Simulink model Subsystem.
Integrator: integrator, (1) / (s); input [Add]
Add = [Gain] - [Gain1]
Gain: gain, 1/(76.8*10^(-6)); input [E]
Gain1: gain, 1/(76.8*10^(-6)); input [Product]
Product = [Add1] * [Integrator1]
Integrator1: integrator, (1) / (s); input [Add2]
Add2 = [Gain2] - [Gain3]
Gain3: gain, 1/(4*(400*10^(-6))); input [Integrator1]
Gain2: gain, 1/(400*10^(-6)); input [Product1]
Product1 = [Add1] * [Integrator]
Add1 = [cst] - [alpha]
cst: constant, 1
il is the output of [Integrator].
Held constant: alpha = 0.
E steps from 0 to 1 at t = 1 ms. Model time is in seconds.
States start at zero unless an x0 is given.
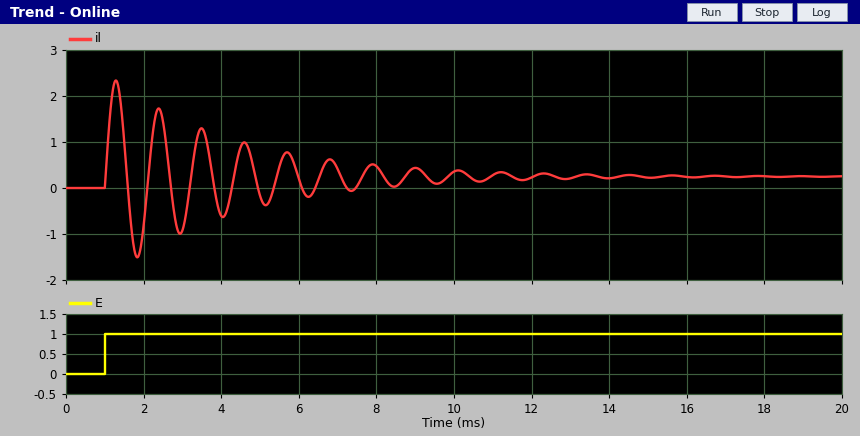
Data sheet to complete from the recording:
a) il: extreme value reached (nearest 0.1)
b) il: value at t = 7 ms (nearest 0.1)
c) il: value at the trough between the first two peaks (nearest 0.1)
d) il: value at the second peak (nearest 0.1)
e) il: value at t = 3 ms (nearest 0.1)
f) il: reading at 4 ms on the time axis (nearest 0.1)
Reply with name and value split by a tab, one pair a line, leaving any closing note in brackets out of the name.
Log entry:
il: extreme value reached	2.3
il: value at t = 7 ms	0.4
il: value at the trough between the first two peaks	-1.5
il: value at the second peak	1.7
il: value at t = 3 ms	-0.9
il: reading at 4 ms on the time axis	-0.6
